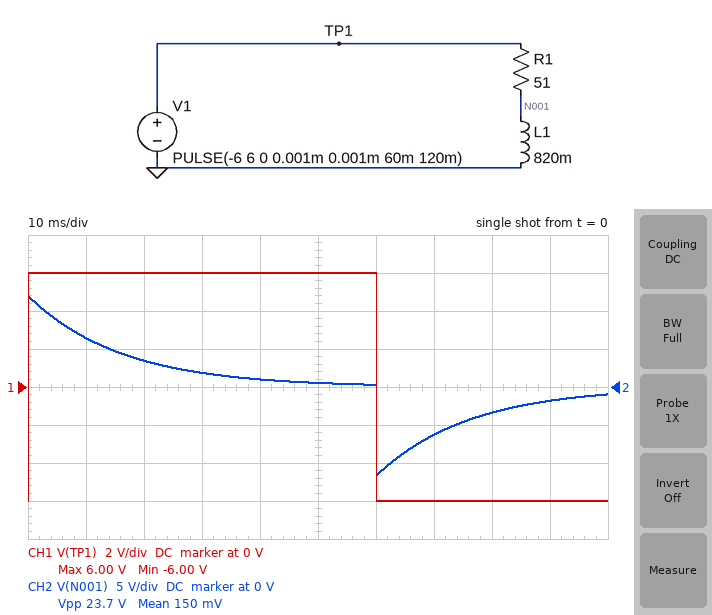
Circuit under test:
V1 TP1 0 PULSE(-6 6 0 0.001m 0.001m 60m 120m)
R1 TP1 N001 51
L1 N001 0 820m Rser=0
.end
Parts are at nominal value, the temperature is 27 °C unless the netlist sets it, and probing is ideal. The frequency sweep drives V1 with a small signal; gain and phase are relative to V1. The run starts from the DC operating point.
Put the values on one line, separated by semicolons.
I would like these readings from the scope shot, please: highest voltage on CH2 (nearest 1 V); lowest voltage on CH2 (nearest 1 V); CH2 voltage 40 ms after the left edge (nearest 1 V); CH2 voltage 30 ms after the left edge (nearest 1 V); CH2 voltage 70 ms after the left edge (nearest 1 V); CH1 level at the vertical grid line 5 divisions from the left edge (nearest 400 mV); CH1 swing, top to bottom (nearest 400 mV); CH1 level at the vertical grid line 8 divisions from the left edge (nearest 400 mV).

12 V; -12 V; 1 V; 2 V; -6 V; 6.0 V; 12.0 V; -6.0 V
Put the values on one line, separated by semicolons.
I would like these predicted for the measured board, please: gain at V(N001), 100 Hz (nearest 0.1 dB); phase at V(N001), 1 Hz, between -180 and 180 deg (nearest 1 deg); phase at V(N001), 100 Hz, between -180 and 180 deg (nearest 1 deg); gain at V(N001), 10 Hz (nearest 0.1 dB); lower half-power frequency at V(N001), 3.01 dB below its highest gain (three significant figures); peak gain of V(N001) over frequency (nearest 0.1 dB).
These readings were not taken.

0 dB; 84 deg; 6 deg; -3.0 dB; 9.90 Hz; 0 dB
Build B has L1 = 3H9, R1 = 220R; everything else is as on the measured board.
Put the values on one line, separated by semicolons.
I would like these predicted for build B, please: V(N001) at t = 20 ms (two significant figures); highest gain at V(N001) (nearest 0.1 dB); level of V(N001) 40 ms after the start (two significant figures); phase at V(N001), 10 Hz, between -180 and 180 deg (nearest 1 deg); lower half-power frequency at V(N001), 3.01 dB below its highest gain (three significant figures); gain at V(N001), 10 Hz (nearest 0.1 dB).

3.9 V; 0 dB; 1.3 V; 42 deg; 8.98 Hz; -2.6 dB
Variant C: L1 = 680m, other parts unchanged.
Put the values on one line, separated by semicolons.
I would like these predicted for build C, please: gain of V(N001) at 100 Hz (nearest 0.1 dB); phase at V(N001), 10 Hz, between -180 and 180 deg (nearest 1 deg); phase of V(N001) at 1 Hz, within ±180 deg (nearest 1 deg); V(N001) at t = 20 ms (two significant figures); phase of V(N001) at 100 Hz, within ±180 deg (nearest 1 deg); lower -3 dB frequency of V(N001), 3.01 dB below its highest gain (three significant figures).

-0.1 dB; 50 deg; 85 deg; 2.7 V; 7 deg; 11.9 Hz
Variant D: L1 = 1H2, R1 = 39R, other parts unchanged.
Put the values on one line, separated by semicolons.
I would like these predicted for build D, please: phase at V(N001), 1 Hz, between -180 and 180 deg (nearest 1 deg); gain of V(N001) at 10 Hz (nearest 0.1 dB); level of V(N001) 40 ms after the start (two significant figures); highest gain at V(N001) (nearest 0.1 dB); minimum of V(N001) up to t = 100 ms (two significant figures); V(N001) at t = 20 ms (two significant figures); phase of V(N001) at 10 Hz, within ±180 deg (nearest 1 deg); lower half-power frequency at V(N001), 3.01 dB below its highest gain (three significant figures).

79 deg; -1.0 dB; 3.3 V; 0 dB; -10 V; 6.3 V; 27 deg; 5.17 Hz
